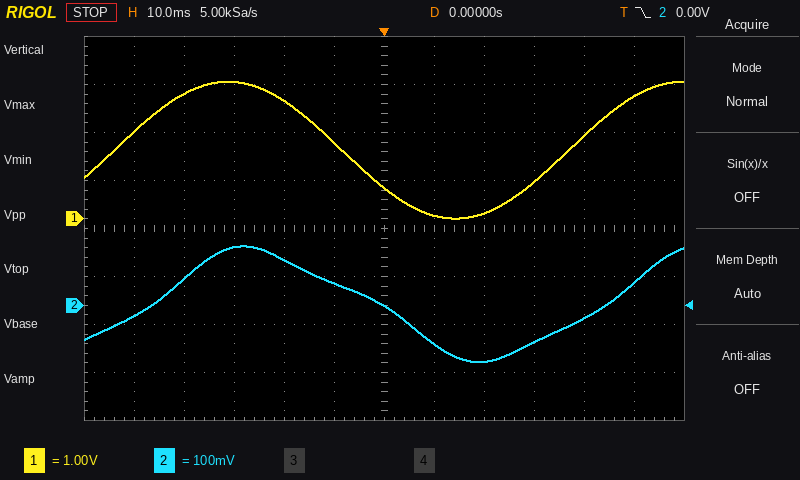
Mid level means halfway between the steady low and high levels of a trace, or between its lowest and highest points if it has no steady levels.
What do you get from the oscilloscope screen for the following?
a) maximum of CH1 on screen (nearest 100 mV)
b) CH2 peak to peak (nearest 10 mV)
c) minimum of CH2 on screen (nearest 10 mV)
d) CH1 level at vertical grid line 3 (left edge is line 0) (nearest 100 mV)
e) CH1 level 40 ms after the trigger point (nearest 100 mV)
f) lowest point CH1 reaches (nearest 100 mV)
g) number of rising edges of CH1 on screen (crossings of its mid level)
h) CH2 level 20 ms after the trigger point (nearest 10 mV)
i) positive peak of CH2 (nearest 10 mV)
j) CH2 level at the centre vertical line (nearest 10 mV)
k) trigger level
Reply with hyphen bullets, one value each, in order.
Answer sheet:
- 2.9 V
- 240 mV
- -120 mV
- 2.9 V
- 1.7 V
- 0.0 V
- 2
- -120 mV
- 120 mV
- 0 mV
- 0.00 V
